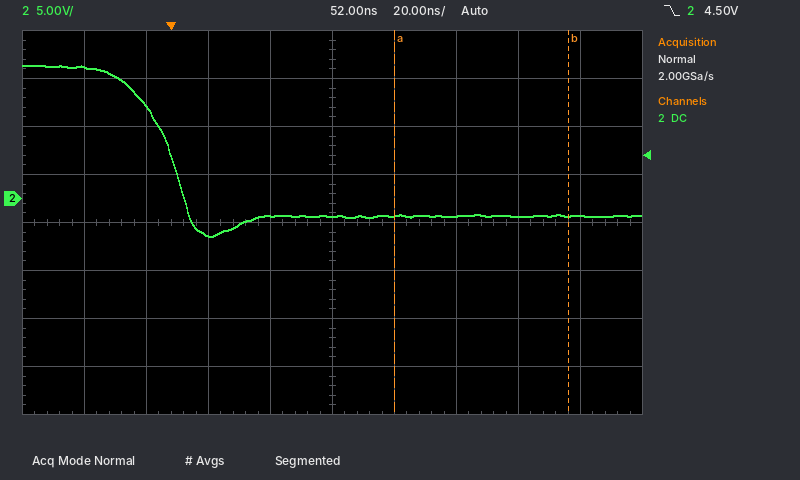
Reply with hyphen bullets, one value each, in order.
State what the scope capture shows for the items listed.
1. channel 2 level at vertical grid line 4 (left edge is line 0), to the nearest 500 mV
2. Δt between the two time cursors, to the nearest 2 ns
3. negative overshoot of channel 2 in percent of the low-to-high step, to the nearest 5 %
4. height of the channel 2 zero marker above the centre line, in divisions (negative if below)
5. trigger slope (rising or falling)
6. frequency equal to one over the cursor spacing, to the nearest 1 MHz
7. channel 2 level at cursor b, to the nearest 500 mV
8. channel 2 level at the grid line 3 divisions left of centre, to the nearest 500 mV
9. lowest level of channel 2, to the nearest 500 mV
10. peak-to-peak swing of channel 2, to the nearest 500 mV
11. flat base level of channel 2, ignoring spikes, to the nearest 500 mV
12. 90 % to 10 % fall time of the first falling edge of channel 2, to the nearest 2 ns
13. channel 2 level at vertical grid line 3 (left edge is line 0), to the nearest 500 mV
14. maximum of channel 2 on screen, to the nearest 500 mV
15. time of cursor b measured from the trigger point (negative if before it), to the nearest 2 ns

- -2.0 V
- 56 ns
- 15 %
- +0.5 div
- falling
- 18 MHz
- -2.0 V
- 9.5 V
- -4.0 V
- 18.0 V
- -2.0 V
- 20 ns
- -4.0 V
- 14.0 V
- +128 ns
